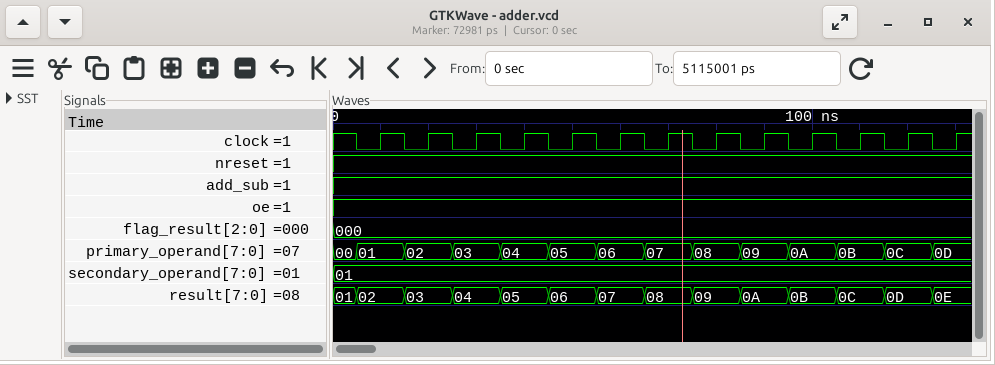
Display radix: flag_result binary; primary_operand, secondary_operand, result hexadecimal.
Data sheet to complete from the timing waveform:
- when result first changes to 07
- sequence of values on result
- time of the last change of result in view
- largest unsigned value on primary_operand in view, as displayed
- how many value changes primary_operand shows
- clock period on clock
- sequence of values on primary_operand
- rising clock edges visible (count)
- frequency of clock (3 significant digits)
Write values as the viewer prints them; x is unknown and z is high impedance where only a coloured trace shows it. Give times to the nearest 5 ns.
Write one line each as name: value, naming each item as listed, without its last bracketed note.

when result first changes to 07: 55 ns
sequence of values on result: 01, 02, 03, 04, 05, 06, 07, 08, 09, 0A, 0B, 0C, 0D, 0E
time of the last change of result in view: 125 ns
largest unsigned value on primary_operand in view, as displayed: 0D
how many value changes primary_operand shows: 13
clock period on clock: 10 ns
sequence of values on primary_operand: 00, 01, 02, 03, 04, 05, 06, 07, 08, 09, 0A, 0B, 0C, 0D
rising clock edges visible: 13
frequency of clock: 100 MHz
